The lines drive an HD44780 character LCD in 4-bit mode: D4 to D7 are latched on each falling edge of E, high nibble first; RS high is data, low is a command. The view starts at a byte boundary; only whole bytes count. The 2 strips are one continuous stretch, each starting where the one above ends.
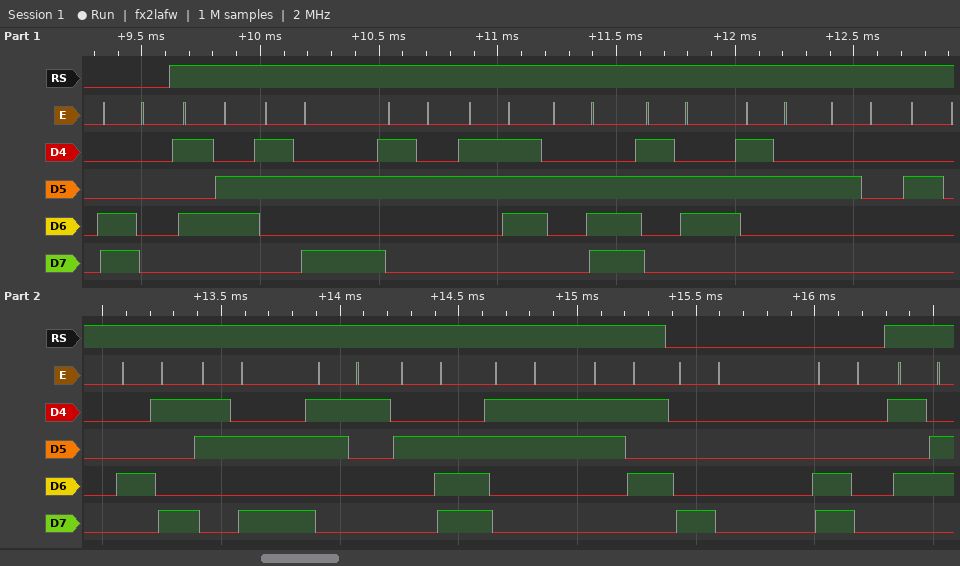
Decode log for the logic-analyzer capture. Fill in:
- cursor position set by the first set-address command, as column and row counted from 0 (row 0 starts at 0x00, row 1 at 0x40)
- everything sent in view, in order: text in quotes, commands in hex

column 0, row 1
0xC0 "V:27.62  I:1.35" 0x80 0xC0 "V"
